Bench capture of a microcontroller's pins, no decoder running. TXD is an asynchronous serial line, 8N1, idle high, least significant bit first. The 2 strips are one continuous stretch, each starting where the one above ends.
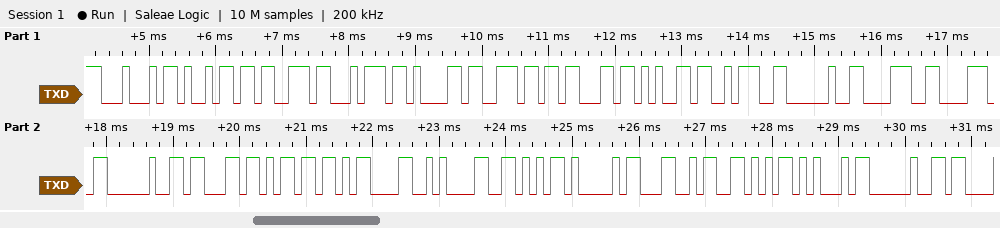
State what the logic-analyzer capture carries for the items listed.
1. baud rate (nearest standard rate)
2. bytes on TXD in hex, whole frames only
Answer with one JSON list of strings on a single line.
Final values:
["9600 baud", "44 69 73 74 61 6E 63 65 3A 20 38 38 20 63 6D 0D 0A 56 41 4C 56 45 20"]
